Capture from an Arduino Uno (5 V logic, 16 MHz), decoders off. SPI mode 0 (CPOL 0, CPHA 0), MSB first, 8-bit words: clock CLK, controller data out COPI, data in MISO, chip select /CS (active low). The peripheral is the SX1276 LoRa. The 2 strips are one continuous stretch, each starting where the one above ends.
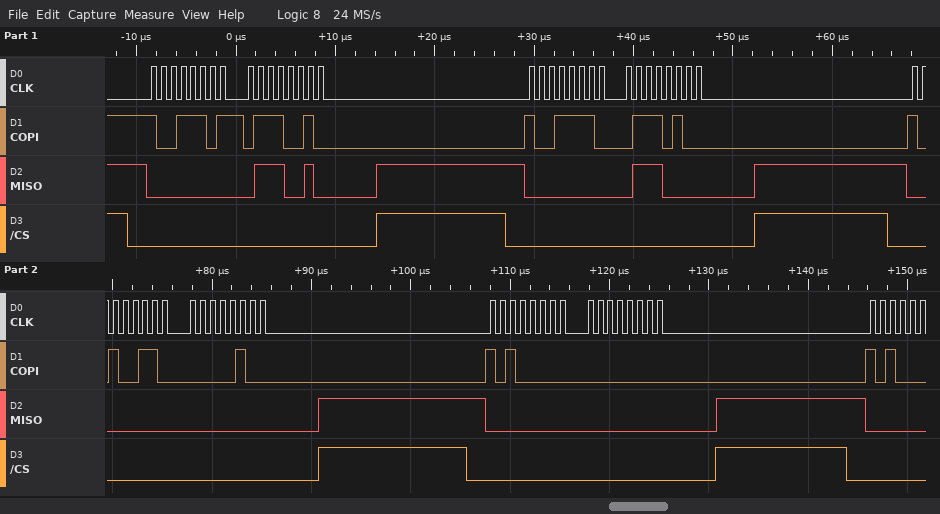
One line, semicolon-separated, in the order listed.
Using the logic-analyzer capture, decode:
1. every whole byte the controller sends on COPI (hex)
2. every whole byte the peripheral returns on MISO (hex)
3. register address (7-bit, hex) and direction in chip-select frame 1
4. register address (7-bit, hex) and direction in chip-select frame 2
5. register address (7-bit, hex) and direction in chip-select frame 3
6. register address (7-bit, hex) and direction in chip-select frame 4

9D 72 9E 74 A6 04 A0 00; 00 72 00 70 00 00 00 00; 0x1D write; 0x1E write; 0x26 write; 0x20 write
